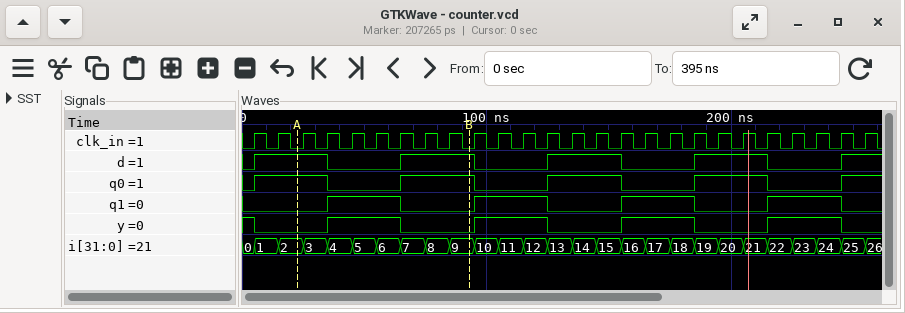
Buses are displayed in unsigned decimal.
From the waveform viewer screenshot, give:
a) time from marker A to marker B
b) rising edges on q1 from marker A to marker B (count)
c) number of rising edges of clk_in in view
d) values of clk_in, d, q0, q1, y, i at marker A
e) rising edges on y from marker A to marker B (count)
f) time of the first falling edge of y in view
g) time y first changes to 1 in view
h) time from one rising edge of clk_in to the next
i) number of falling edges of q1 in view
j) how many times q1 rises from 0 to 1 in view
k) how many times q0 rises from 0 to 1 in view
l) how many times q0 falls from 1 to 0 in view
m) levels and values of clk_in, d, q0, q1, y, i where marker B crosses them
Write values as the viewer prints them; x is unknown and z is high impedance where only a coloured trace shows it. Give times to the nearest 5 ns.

70 ns
1
26
clk_in=0, d=1, q0=1, q1=0, y=0, i=2
1
5 ns
35 ns
10 ns
4
4
5
4
clk_in=0, d=1, q0=1, q1=0, y=0, i=9
